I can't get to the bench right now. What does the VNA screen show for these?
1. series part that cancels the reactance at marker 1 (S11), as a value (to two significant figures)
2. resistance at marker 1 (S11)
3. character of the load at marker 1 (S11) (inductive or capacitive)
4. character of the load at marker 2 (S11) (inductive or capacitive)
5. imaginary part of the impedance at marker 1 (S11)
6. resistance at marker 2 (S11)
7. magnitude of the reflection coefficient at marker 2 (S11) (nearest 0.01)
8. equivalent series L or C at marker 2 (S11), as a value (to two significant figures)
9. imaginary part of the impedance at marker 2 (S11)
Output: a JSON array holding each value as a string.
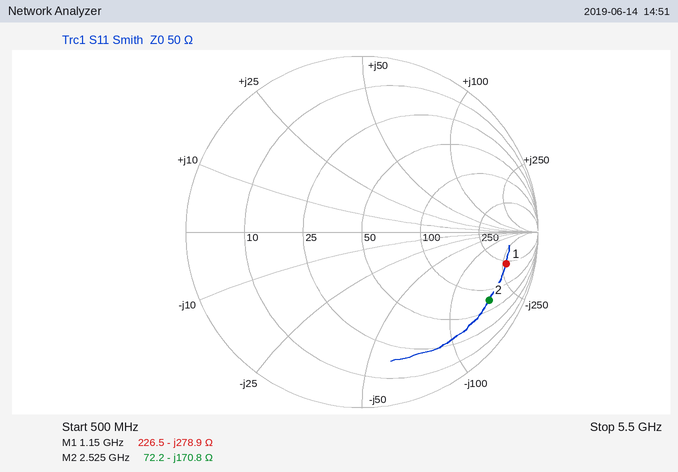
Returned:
["39 nH", "226.5 Ω", "capacitive", "capacitive", "-278.9 Ω", "72.2 Ω", "0.82", "370 fF", "-170.8 Ω"]
